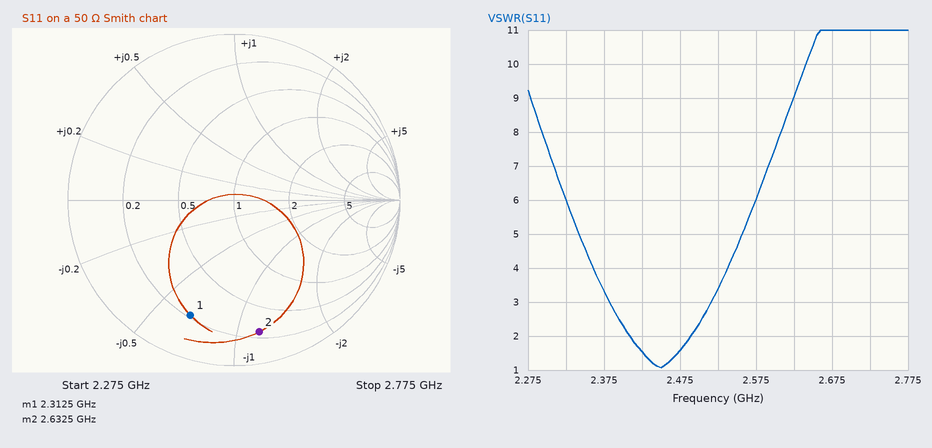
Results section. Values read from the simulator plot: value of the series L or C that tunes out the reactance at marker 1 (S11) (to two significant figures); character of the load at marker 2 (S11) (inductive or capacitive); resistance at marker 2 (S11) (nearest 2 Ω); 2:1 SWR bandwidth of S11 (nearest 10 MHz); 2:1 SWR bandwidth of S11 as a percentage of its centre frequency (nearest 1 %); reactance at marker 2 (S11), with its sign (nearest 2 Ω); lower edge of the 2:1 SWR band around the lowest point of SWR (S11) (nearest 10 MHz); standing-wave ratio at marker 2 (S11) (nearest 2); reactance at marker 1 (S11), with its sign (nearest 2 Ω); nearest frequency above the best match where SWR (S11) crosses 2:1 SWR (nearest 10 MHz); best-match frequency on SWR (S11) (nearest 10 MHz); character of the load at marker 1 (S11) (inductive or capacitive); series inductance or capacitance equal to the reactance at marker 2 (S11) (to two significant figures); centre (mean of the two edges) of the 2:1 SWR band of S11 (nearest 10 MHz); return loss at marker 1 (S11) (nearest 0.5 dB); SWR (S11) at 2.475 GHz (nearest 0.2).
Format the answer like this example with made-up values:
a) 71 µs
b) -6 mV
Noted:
a) 2.3 nH
b) capacitive
c) 12 Ω
d) 80 MHz
e) 3 %
f) -58 Ω
g) 2.41 GHz
h) 10
i) -34 Ω
j) 2.49 GHz
k) 2.45 GHz
l) capacitive
m) 1.0 pF
n) 2.45 GHz
o) 2.5 dB
p) 1.6
